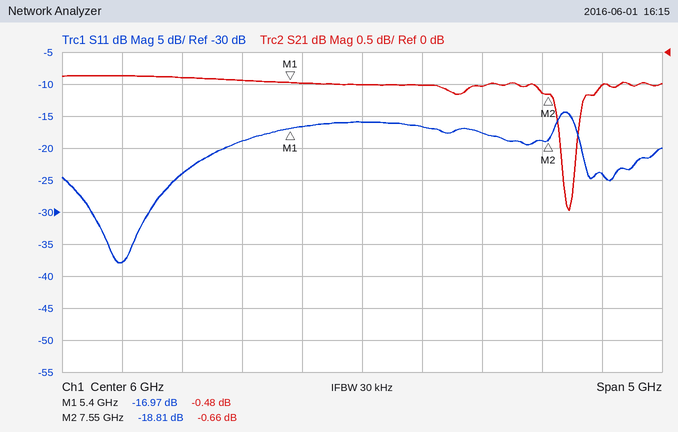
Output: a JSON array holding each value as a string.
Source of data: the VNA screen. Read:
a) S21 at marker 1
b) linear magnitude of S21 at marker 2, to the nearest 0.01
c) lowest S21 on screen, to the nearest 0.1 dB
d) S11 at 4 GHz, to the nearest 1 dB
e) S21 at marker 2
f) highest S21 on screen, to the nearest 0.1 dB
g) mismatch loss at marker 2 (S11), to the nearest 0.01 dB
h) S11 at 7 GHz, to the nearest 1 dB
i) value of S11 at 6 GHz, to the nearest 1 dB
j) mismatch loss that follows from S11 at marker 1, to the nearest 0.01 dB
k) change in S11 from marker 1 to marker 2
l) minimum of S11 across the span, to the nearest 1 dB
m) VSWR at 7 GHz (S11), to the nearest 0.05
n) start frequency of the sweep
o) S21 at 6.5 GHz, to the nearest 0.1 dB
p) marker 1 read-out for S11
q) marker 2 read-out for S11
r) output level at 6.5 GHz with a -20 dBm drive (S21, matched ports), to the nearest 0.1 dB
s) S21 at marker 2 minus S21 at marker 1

["-0.48 dB", "0.93", "-2.5 dB", "-38 dB", "-0.66 dB", "-0.4 dB", "0.06 dB", "-18 dB", "-16 dB", "0.09 dB", "-1.84 dB", "-38 dB", "1.30", "3.5 GHz", "-0.5 dB", "-16.97 dB", "-18.81 dB", "-20.5 dBm", "-0.18 dB"]
